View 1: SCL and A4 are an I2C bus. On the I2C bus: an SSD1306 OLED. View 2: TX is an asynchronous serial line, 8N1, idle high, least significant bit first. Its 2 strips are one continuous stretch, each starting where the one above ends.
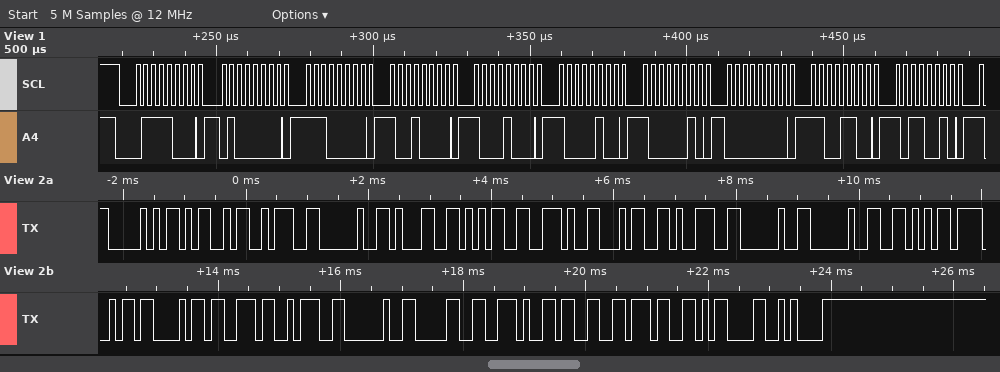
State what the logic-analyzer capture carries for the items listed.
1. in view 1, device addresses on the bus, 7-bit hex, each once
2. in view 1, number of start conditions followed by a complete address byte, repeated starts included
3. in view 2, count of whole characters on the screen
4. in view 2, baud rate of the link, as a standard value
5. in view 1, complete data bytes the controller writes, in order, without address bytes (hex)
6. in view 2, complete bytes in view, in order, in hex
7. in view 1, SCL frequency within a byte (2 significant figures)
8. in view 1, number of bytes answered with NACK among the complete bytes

0x3C
1
23
9600 baud
40 E0 90 88 84 82 00 CC B2
0x50 0x4D 0x3A 0x20 0x31 0x35 0x2E 0x34 0x39 0x20 0x20 0x56 0x4F 0x43 0x73 0x3A 0x20 0x30 0x2E 0x33 0x37 0x0D 0x0A
400 kHz
0
